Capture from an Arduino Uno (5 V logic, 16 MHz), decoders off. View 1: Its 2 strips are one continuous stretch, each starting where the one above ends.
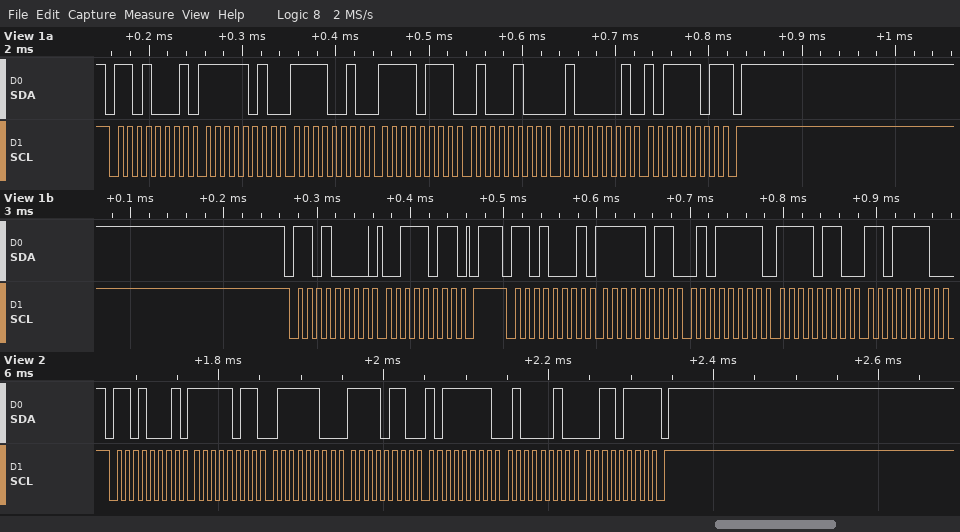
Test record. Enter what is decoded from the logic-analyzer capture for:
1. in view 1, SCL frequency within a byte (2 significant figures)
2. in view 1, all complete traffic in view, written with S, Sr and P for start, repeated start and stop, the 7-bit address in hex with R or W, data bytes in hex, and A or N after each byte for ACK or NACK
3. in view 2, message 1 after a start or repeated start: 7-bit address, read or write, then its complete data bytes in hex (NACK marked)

100 kHz
S 68R A FA A F2 A F7 A 44 A 41 A BD N P S 68W A 3B A P S 68R A FB A 5F A F6 A DE A
0x68 read: FB 7C F6 BF 42 37 NACK
